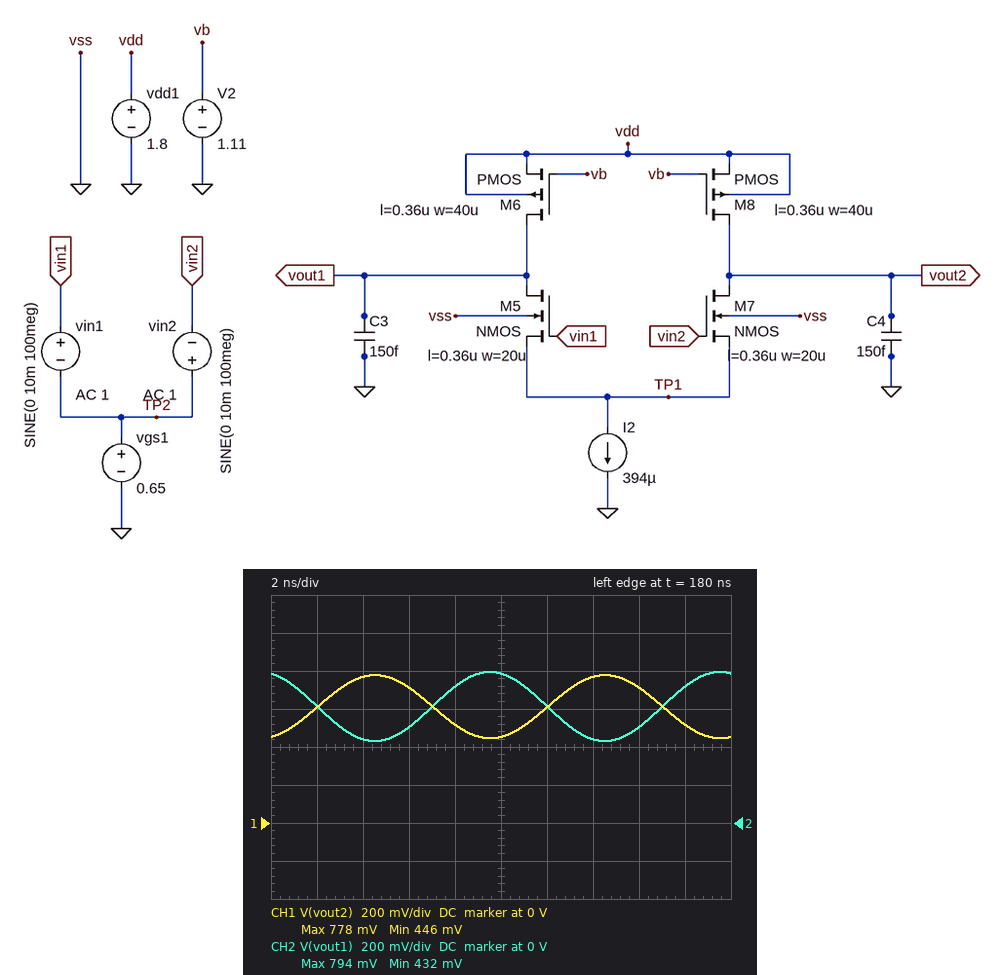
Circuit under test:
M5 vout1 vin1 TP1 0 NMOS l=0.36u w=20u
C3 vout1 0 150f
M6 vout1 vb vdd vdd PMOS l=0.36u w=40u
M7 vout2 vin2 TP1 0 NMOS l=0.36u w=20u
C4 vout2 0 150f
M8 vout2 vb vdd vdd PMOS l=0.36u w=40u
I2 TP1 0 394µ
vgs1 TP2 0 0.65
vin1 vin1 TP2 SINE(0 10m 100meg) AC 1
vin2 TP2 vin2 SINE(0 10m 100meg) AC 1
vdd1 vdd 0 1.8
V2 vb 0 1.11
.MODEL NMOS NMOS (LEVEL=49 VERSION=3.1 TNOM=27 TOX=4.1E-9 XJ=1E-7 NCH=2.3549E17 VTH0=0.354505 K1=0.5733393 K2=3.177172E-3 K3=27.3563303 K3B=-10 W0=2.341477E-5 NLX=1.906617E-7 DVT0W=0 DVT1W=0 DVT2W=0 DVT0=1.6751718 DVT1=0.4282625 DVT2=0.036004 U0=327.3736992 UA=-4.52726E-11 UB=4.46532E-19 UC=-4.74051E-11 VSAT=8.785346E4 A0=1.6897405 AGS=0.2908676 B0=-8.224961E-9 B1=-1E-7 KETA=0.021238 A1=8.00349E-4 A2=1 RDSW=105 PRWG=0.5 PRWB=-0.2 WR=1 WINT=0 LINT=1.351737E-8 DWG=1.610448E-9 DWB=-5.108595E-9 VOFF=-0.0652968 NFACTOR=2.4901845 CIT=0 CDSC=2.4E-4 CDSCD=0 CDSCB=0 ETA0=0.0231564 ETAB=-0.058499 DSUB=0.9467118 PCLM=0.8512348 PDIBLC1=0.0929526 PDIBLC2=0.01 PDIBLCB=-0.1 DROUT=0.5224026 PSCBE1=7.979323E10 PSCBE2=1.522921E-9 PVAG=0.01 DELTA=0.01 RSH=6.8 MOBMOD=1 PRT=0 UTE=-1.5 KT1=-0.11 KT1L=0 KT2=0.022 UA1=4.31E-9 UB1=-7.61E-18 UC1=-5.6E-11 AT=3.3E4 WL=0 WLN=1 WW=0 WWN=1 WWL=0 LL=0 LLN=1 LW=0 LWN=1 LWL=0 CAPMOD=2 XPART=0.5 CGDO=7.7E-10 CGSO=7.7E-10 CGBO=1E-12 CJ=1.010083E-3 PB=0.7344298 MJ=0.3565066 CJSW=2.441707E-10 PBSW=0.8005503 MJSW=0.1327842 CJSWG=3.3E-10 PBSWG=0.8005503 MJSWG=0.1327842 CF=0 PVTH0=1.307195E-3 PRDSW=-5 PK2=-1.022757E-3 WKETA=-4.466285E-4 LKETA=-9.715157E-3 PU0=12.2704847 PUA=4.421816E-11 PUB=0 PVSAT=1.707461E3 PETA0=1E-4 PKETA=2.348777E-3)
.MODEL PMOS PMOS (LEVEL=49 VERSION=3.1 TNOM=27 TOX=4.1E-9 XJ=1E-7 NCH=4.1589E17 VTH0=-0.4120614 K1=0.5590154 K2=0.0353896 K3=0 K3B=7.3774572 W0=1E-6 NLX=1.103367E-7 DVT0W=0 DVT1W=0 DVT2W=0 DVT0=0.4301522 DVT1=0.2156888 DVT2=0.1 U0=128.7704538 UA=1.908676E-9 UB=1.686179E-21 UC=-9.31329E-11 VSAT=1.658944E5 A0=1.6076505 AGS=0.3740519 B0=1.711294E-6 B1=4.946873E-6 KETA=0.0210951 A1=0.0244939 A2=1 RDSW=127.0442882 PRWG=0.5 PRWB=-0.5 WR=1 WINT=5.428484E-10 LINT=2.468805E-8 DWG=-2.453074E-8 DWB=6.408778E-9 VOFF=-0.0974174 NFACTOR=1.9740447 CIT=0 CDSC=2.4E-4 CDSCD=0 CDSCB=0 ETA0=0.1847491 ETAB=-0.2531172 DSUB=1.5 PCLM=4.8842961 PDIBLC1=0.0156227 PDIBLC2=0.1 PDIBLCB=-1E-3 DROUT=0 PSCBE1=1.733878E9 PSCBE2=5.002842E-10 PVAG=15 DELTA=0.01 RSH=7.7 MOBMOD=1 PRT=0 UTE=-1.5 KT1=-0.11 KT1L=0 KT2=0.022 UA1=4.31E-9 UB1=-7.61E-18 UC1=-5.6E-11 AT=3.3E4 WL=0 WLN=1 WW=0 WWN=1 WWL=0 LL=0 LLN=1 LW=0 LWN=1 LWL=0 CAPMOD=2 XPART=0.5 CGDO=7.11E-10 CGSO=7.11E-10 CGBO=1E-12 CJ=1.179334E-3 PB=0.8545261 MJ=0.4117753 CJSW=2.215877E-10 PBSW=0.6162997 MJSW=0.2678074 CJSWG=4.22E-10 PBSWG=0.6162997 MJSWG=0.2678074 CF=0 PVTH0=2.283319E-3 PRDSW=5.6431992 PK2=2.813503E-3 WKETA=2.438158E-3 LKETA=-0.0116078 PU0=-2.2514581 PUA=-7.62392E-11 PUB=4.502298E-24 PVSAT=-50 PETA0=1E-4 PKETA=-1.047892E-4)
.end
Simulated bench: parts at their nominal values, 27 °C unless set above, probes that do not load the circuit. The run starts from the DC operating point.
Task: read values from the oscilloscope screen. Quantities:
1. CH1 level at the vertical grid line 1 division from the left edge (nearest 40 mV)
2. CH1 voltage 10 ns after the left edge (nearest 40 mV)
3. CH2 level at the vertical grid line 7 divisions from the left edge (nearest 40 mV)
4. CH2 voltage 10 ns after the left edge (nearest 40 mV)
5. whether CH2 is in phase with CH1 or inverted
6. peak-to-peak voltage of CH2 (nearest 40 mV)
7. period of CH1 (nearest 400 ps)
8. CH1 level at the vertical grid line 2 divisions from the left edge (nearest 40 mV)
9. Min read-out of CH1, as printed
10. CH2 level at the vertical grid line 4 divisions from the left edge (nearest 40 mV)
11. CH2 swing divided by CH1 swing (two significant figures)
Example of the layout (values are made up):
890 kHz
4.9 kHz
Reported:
600 mV
440 mV
440 mV
800 mV
inverted
360 mV
10.0 ns
760 mV
446 mV
720 mV
1.1
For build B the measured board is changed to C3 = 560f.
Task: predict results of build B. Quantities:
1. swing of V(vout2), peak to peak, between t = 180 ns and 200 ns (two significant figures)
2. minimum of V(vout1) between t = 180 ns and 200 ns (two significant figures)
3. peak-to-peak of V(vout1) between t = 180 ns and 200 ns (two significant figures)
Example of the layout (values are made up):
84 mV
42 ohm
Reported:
340 mV
550 mV
120 mV
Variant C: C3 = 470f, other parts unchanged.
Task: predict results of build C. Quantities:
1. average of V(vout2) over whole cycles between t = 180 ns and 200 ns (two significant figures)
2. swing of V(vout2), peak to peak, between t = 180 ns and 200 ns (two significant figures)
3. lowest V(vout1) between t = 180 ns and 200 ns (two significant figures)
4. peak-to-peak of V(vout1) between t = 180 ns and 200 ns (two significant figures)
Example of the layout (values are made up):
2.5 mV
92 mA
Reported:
610 mV
340 mV
540 mV
140 mV
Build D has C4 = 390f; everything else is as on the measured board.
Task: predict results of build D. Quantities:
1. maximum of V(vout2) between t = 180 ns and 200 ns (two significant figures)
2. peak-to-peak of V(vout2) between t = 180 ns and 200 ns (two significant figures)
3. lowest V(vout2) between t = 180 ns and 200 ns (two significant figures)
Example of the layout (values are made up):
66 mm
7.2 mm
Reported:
690 mV
160 mV
530 mV
